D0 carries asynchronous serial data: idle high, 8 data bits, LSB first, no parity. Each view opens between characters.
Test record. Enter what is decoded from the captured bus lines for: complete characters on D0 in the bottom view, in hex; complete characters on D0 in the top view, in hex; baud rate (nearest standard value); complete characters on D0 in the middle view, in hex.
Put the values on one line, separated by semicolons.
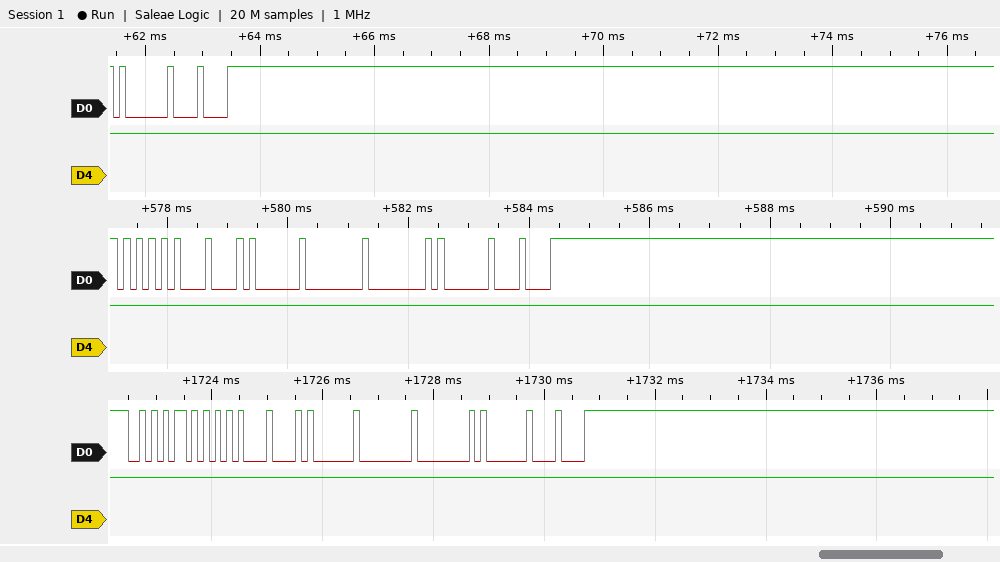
AA, 55, 08, 01, 00, 00, 01, 08; 01, 08; 9600 baud; 55, 08, 01, 00, 00, 01, 08
